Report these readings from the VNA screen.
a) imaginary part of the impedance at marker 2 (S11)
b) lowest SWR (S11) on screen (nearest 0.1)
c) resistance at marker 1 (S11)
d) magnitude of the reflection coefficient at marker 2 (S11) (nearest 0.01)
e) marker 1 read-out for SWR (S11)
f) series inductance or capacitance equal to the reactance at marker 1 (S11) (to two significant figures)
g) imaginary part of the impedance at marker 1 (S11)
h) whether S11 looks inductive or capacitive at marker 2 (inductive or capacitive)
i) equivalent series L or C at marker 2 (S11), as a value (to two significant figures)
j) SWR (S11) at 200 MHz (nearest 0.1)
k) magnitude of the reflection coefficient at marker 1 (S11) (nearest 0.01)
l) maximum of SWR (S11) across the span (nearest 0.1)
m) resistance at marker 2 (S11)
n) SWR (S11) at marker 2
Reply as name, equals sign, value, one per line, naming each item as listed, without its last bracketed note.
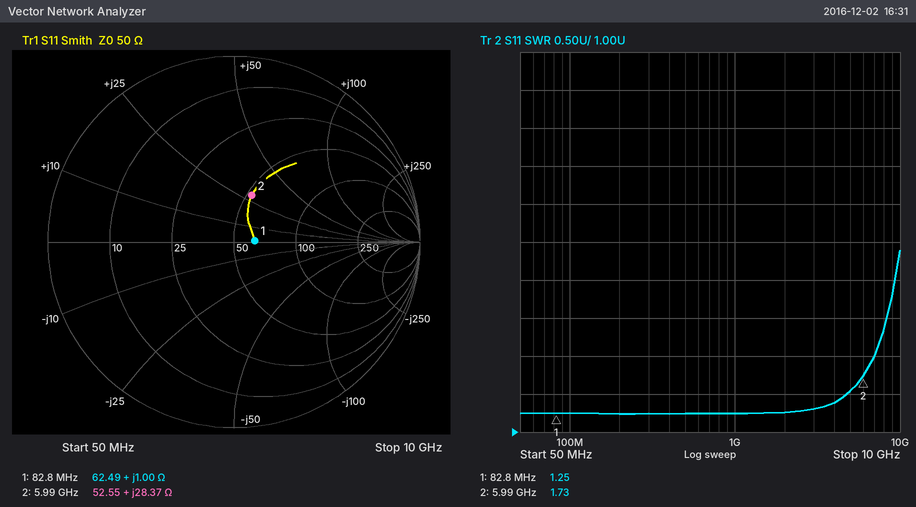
imaginary part of the impedance at marker 2 = +28.37 Ω
lowest SWR (S11) on screen = 1.2
resistance at marker 1 = 62.49 Ω
magnitude of the reflection coefficient at marker 2 (S11) = 0.27
marker 1 read-out for SWR = 1.25
series inductance or capacitance equal to the reactance at marker 1 (S11) = 1.9 nH
imaginary part of the impedance at marker 1 = +1.00 Ω
whether S11 looks inductive or capacitive at marker 2 = inductive
equivalent series L or C at marker 2 (S11), as a value = 750 pH
SWR (S11) at 200 MHz = 1.2
magnitude of the reflection coefficient at marker 1 (S11) = 0.11
maximum of SWR (S11) across the span = 3.4
resistance at marker 2 = 52.55 Ω
SWR (S11) at marker 2 = 1.73
